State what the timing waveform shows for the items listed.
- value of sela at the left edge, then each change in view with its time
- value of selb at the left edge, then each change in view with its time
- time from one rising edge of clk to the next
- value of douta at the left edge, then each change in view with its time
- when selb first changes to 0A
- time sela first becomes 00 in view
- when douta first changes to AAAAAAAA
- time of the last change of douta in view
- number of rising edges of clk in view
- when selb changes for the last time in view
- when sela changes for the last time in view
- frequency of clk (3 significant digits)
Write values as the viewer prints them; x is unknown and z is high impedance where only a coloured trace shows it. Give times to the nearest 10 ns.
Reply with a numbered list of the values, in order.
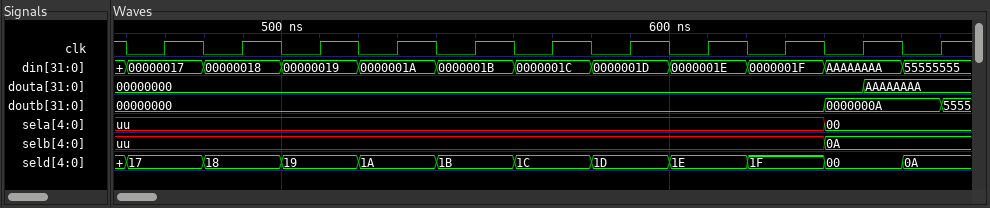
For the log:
1. uu, 00 at 640 ns
2. uu, 0A at 640 ns
3. 20 ns
4. 00000000, AAAAAAAA at 650 ns
5. 640 ns
6. 640 ns
7. 650 ns
8. 650 ns
9. 11
10. 640 ns
11. 640 ns
12. 50.0 MHz
